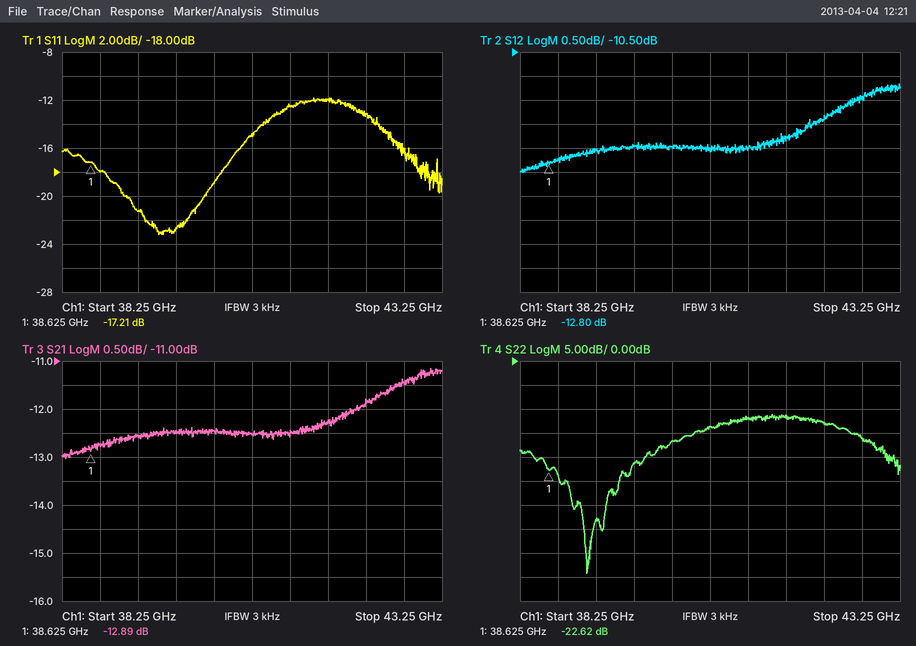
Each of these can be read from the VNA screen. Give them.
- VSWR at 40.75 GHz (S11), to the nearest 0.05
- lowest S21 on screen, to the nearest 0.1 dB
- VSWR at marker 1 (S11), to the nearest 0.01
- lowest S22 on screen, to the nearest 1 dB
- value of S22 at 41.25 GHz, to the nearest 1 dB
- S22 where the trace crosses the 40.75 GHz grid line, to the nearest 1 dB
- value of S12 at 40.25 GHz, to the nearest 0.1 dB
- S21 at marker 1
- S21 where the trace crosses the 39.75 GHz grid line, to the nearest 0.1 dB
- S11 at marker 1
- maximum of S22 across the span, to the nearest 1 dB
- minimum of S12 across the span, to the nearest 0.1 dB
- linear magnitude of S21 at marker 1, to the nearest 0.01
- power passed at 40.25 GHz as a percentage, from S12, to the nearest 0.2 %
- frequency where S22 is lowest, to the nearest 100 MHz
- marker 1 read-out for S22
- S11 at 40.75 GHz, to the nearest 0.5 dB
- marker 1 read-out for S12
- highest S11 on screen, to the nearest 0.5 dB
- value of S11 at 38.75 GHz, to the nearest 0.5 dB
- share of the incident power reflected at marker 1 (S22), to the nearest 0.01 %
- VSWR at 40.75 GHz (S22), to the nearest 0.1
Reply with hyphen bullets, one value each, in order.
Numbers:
- 1.45
- -13.0 dB
- 1.32
- -44 dB
- -12 dB
- -14 dB
- -12.5 dB
- -12.89 dB
- -12.5 dB
- -17.21 dB
- -11 dB
- -13.0 dB
- 0.23
- 5.6 %
- 39.1 GHz
- -22.62 dB
- -15.0 dB
- -12.80 dB
- -12.0 dB
- -18.0 dB
- 0.55 %
- 1.5
